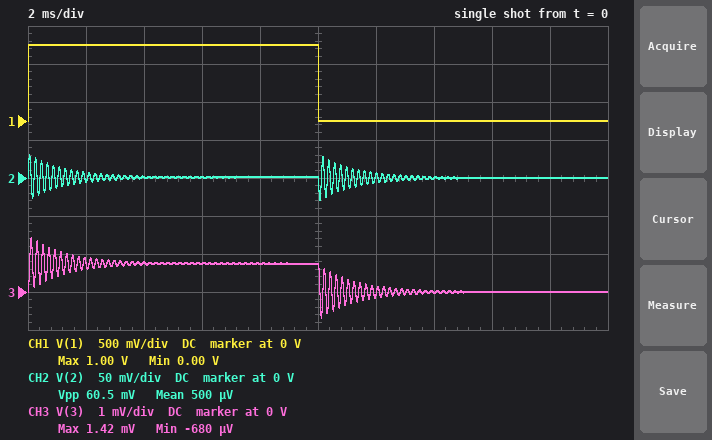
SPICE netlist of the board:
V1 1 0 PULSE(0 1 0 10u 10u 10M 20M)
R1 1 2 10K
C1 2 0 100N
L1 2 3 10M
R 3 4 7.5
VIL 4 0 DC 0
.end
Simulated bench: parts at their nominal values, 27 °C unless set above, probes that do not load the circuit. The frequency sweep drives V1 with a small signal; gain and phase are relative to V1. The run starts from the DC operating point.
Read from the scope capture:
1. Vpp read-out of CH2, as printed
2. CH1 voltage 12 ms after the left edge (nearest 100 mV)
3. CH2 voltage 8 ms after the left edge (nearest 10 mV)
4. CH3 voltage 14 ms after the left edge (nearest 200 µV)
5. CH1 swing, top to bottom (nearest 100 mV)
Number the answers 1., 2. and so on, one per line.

1. 60.5 mV
2. 0 V
3. 0 V
4. 0 V
5. 1.0 V
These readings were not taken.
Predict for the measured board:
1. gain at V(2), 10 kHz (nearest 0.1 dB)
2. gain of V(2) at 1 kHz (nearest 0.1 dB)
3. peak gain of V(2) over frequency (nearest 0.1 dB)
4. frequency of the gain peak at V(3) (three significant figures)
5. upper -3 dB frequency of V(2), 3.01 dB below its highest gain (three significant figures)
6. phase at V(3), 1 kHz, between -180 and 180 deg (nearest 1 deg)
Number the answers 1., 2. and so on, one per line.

1. -33.4 dB
2. -43.6 dB
3. -4.9 dB
4. 5.03 kHz
5. 5.18 kHz
6. -1 deg
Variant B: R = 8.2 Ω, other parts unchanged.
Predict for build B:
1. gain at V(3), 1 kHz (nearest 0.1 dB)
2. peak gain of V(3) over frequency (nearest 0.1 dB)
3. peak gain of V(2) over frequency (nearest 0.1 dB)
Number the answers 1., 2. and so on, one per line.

1. -61.4 dB
2. -36.9 dB
3. -5.2 dB
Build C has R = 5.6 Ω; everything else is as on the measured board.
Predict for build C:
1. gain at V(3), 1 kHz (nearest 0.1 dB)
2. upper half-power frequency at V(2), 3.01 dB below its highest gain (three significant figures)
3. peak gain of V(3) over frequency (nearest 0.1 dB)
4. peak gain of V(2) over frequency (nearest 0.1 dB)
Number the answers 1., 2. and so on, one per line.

1. -64.7 dB
2. 5.16 kHz
3. -38.9 dB
4. -3.9 dB
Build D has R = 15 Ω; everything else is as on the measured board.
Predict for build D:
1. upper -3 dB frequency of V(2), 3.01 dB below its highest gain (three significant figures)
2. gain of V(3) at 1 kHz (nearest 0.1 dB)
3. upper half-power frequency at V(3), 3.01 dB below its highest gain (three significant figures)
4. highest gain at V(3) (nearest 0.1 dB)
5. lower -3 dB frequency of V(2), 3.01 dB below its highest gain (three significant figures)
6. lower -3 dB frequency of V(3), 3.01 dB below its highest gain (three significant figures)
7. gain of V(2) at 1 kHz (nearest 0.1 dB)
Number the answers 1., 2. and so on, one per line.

1. 5.24 kHz
2. -56.1 dB
3. 5.22 kHz
4. -34.4 dB
5. 4.84 kHz
6. 4.83 kHz
7. -43.5 dB
